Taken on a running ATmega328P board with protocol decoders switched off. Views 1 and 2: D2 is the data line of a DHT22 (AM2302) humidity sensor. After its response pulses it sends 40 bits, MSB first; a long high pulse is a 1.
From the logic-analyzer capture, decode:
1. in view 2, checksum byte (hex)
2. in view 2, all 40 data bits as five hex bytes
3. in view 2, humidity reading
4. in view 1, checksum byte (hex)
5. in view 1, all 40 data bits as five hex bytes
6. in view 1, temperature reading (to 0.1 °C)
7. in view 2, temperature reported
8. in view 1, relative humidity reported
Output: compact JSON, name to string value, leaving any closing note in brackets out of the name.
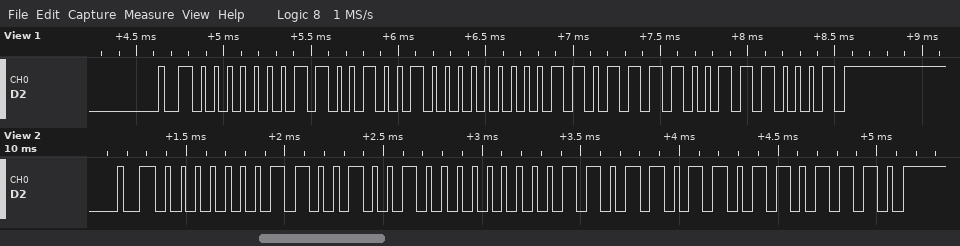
{"in view 2, checksum byte": "0x6E", "in view 2, all 40 data bits as five hex bytes": "01 92 00 DB 6E", "in view 2, humidity reading": "40.2 %", "in view 1, checksum byte": "0x71", "in view 1, all 40 data bits as five hex bytes": "01 92 00 DE 71", "in view 1, temperature reading": "22.2 °C", "in view 2, temperature reported": "21.9 °C", "in view 1, relative humidity reported": "40.2 %"}
